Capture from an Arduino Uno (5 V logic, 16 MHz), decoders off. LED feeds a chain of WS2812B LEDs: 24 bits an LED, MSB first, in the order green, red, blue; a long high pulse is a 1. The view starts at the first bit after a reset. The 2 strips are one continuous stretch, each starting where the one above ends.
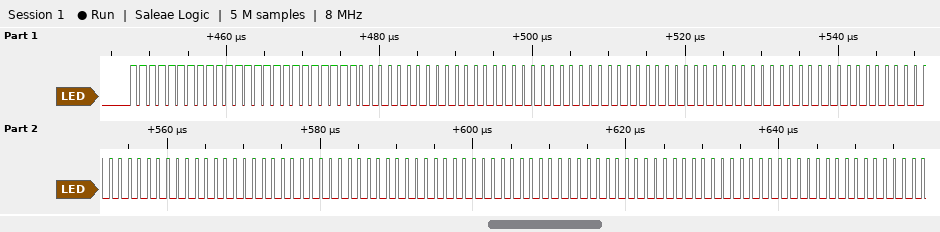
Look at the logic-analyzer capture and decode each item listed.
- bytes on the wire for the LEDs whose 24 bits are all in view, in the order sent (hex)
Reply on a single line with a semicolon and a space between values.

FF FF FF 00 00 00 00 00 00 00 00 00 00 00 00 00 00 00 00 00 00
